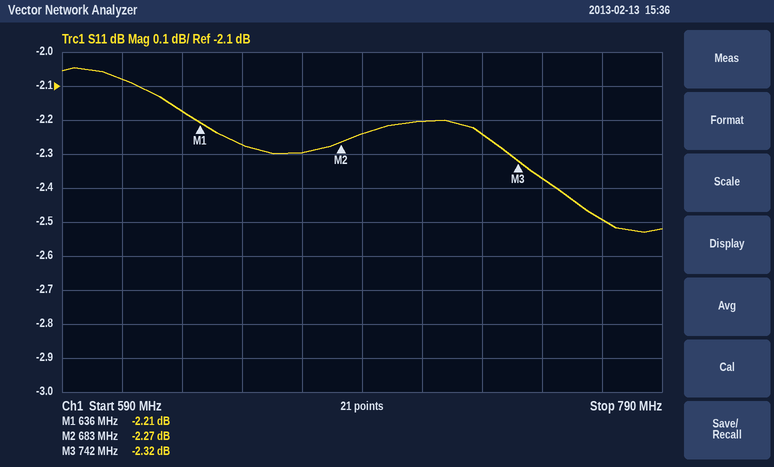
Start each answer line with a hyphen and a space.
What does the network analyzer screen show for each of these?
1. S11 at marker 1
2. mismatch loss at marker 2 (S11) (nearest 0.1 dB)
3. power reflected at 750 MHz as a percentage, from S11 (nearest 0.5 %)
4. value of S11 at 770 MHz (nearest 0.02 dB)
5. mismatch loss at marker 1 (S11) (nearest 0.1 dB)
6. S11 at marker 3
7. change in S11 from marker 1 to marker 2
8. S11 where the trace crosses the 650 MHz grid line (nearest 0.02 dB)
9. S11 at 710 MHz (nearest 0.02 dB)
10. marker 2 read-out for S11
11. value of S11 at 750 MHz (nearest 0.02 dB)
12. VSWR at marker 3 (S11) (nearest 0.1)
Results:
- -2.21 dB
- 3.9 dB
- 58.0 %
- -2.50 dB
- 4.0 dB
- -2.32 dB
- -0.06 dB
- -2.28 dB
- -2.20 dB
- -2.27 dB
- -2.38 dB
- 7.5
